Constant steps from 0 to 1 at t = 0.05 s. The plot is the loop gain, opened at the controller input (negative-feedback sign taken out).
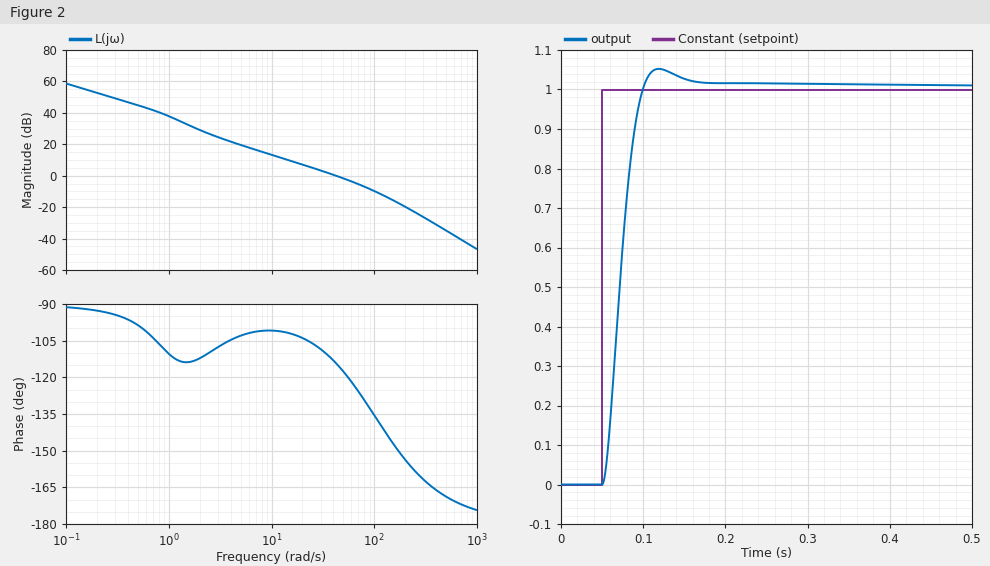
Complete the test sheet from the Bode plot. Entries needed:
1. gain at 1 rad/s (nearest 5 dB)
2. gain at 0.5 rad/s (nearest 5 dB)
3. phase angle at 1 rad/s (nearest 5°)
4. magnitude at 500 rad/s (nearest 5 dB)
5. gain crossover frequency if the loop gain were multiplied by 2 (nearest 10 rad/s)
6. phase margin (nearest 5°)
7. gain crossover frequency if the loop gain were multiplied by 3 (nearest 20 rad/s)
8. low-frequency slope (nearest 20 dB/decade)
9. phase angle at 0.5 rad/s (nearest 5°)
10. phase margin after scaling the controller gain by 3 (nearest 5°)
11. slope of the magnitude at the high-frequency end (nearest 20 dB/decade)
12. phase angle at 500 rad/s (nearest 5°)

40 dB
45 dB
-110°
-35 dB
70 rad/s
65°
100 rad/s
-20 dB/decade
-100°
45°
-40 dB/decade
-170°
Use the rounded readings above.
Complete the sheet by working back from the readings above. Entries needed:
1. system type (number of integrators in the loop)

1
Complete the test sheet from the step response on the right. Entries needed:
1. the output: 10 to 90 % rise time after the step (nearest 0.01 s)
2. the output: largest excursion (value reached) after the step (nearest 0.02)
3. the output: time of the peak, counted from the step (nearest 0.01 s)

0.03 s
1.06
0.07 s
